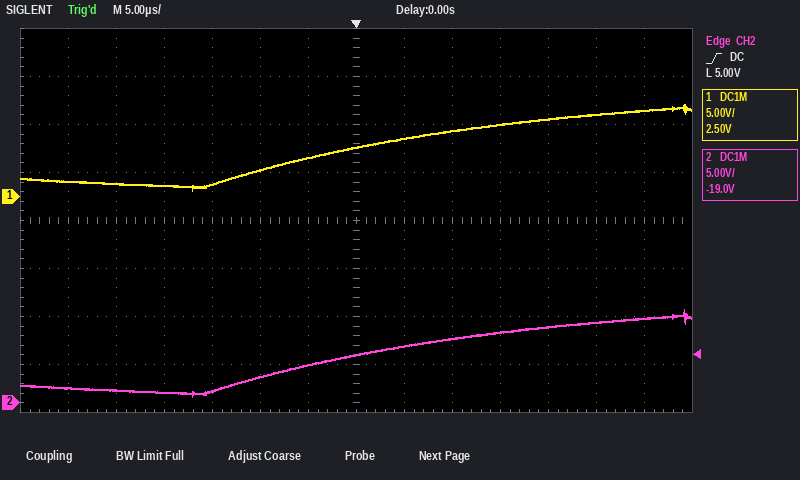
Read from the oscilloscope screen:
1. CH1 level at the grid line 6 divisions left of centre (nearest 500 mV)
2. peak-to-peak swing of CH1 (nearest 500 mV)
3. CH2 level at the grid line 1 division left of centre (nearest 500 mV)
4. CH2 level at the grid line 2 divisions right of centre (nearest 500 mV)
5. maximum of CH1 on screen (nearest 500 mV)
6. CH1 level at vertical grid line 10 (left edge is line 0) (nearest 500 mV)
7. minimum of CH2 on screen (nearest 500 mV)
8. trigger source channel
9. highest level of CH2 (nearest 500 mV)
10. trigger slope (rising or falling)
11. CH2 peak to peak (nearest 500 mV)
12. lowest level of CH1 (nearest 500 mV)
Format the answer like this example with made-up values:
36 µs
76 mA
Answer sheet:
1.5 V
9.0 V
4.0 V
6.5 V
9.5 V
7.5 V
500 mV
CH2
9.5 V
rising
9.0 V
500 mV
